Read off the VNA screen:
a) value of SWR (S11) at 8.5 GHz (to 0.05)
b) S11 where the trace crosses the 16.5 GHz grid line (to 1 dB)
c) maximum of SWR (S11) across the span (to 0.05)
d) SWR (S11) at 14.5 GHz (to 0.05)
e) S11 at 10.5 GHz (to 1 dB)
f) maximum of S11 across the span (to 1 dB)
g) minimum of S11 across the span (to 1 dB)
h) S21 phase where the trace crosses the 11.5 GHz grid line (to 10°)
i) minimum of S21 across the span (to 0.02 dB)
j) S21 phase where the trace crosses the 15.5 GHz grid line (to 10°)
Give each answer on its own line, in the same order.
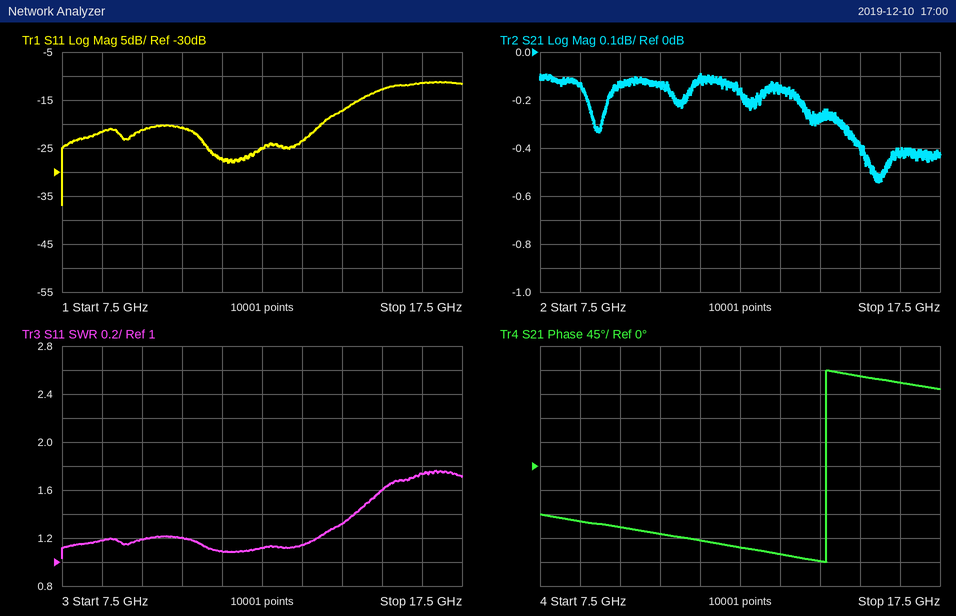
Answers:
1.20
-11 dB
1.75
1.30
-21 dB
-11 dB
-37 dB
-140°
-0.54 dB
170°
